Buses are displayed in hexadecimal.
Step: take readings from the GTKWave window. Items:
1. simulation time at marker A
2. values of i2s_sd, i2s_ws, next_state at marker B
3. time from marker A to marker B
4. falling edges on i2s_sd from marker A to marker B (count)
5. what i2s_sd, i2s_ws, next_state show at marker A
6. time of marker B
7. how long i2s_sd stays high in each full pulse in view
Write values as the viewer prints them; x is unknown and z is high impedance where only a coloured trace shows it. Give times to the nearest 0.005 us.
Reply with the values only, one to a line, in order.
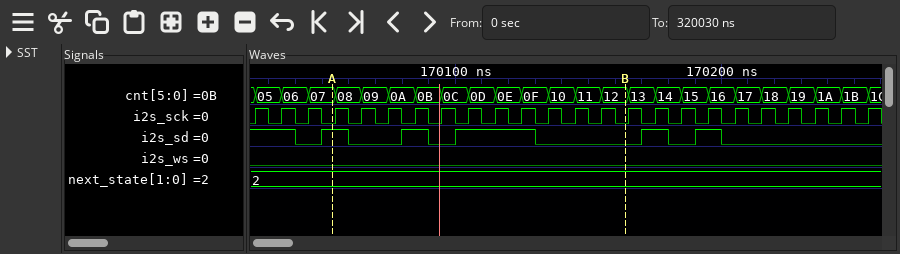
170.055 us
i2s_sd=0, i2s_ws=0, next_state=2
0.11 us
3
i2s_sd=1, i2s_ws=0, next_state=2
170.165 us
0.01 us, 0.01 us, 0.03 us, 0.01 us, 0.01 us
